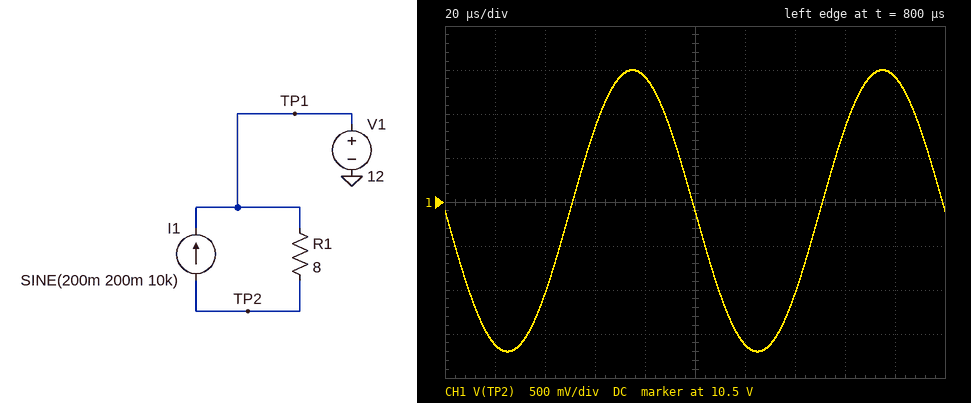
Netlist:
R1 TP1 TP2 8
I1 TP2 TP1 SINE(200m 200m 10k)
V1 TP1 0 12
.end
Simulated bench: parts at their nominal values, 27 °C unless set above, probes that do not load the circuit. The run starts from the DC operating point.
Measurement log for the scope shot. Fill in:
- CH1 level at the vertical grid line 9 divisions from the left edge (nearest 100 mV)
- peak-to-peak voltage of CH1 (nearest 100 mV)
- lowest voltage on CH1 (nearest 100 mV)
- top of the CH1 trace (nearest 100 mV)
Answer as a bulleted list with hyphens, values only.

- 11.9 V
- 3.2 V
- 8.8 V
- 12.0 V
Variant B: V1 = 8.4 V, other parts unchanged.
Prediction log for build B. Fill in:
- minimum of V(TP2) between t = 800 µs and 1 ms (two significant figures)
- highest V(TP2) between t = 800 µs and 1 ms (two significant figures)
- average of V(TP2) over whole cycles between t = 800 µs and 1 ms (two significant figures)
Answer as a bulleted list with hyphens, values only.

- 5.2 V
- 8.4 V
- 6.8 V
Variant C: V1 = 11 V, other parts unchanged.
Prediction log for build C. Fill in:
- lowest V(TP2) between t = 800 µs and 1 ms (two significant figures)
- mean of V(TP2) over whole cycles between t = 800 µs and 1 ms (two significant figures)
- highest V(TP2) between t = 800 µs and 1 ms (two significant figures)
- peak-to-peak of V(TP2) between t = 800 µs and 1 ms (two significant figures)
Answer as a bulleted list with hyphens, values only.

- 7.8 V
- 9.4 V
- 11 V
- 3.2 V
